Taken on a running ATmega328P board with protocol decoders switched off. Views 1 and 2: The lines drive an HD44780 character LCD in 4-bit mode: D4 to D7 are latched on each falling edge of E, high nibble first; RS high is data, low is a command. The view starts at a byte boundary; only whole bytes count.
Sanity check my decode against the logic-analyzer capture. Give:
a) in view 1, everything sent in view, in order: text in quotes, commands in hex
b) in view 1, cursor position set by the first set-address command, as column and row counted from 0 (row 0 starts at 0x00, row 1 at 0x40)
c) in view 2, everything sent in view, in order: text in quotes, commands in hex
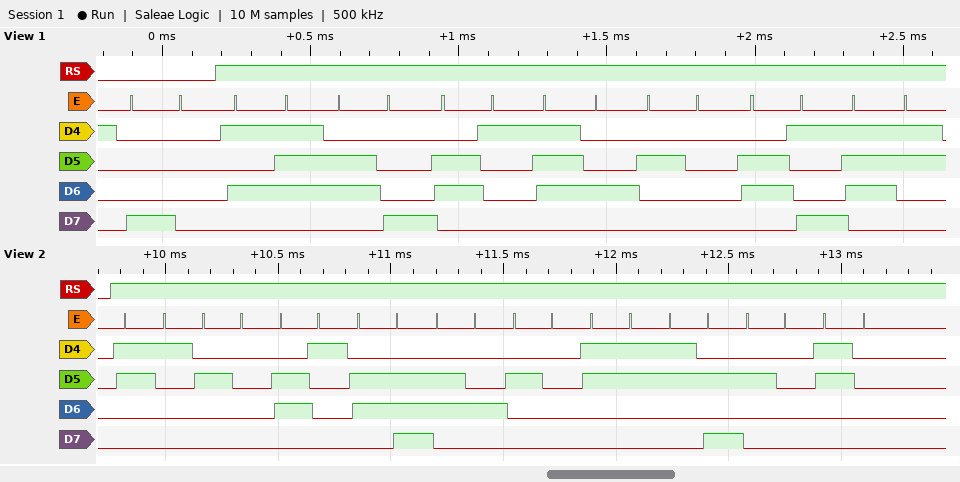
0x80 "What is"
column 0, row 0
"1 and 3: 0"
